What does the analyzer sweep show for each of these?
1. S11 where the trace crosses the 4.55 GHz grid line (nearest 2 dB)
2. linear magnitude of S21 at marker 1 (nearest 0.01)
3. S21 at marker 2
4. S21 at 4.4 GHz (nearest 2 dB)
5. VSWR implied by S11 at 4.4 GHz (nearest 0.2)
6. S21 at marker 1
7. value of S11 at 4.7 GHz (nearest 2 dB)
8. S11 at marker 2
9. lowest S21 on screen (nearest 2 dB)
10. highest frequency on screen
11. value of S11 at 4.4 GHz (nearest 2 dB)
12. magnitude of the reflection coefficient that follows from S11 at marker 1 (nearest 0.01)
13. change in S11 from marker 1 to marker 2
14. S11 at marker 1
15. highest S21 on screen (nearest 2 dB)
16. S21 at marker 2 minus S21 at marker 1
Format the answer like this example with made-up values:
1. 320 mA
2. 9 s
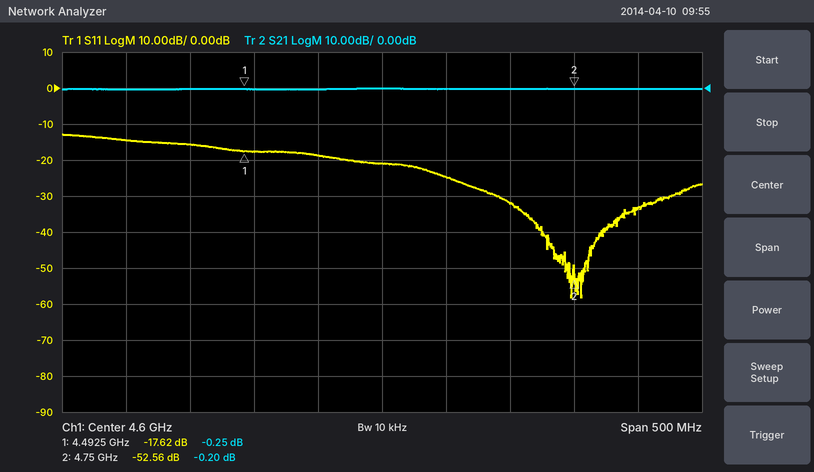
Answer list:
1. -18 dB
2. 0.97
3. -0.20 dB
4. 0 dB
5. 1.4
6. -0.25 dB
7. -32 dB
8. -52.56 dB
9. 0 dB
10. 4.85 GHz
11. -14 dB
12. 0.13
13. -34.94 dB
14. -17.62 dB
15. 0 dB
16. 0.05 dB
